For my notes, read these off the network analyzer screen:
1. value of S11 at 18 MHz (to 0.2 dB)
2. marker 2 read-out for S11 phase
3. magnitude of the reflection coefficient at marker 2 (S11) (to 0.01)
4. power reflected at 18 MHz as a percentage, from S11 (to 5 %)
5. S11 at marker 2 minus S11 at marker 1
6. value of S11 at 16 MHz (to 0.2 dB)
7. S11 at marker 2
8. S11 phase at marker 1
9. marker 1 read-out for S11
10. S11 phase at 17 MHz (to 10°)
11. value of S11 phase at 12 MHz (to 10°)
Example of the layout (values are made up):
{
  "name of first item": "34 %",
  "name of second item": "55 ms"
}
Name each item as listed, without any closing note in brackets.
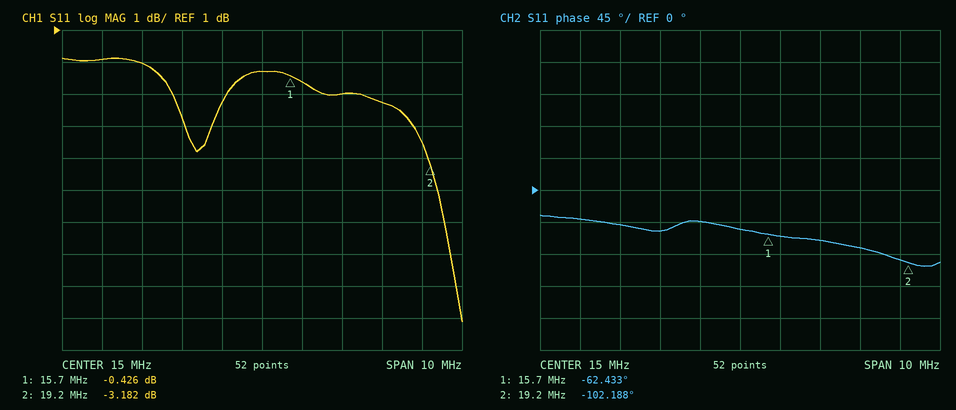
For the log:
{
  "value of S11 at 18 MHz": "-1.2 dB",
  "marker 2 read-out for S11 phase": "-102.188°",
  "magnitude of the reflection coefficient at marker 2 (S11)": "0.69",
  "power reflected at 18 MHz as a percentage, from S11": "75 %",
  "S11 at marker 2 minus S11 at marker 1": "-2.756 dB",
  "value of S11 at 16 MHz": "-0.6 dB",
  "S11 at marker 2": "-3.182 dB",
  "S11 phase at marker 1": "-62.433°",
  "marker 1 read-out for S11": "-0.426 dB",
  "S11 phase at 17 MHz": "-70°",
  "value of S11 phase at 12 MHz": "-50°"
}
